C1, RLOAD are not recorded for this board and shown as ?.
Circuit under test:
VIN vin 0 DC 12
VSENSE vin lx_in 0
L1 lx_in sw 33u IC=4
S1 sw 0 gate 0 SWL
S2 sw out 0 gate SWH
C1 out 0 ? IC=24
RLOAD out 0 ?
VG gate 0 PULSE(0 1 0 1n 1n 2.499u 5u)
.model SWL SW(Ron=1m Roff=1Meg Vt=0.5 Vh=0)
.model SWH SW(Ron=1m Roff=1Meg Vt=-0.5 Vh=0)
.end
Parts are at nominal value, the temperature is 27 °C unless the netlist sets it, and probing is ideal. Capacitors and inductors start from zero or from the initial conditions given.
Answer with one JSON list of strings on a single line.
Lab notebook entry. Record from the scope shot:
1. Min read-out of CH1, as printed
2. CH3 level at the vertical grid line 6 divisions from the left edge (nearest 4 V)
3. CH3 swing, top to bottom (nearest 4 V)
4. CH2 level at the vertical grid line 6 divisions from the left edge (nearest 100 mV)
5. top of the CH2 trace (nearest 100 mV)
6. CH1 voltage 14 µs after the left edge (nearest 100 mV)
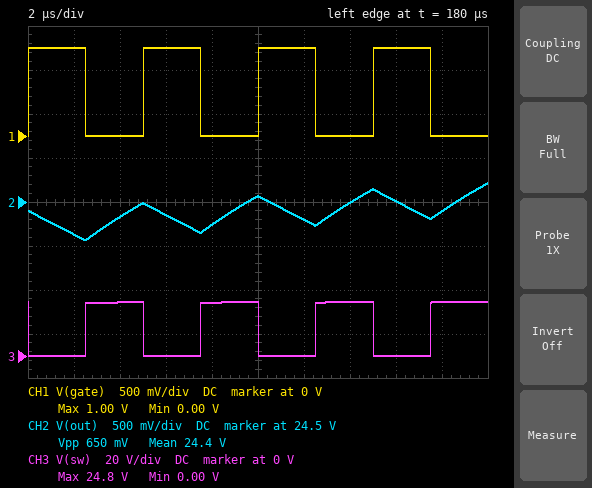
["0.00 V", "0 V", "24 V", "24.3 V", "24.7 V", "0 V"]
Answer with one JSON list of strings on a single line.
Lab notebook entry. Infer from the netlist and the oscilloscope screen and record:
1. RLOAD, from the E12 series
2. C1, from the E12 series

["8.2 Ω", "22 µF"]
